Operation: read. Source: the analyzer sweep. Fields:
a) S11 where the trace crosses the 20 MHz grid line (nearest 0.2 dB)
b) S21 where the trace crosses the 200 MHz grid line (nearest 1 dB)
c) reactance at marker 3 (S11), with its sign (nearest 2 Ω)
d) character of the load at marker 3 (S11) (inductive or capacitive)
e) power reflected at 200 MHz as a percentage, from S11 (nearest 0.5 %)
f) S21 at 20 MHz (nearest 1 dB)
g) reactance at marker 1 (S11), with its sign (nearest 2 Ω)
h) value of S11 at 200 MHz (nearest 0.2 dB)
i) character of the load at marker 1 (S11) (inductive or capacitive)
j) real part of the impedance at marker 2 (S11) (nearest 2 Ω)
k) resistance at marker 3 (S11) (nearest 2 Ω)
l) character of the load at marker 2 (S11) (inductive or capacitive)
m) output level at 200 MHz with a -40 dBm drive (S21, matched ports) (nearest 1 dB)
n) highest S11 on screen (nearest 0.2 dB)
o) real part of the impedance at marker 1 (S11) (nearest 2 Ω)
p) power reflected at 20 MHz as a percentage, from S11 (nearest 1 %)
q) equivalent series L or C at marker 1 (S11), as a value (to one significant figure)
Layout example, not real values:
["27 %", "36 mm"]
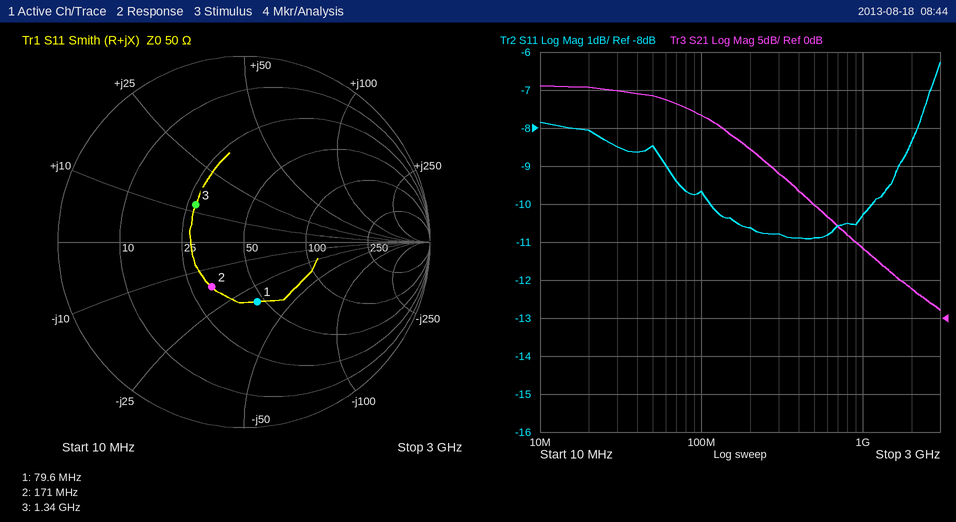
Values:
["-8.0 dB", "22 dB", "+12 Ω", "inductive", "8.5 %", "30 dB", "-34 Ω", "-10.6 dB", "capacitive", "32 Ω", "28 Ω", "capacitive", "-18 dBm", "-6.2 dB", "46 Ω", "16 %", "60 pF"]
